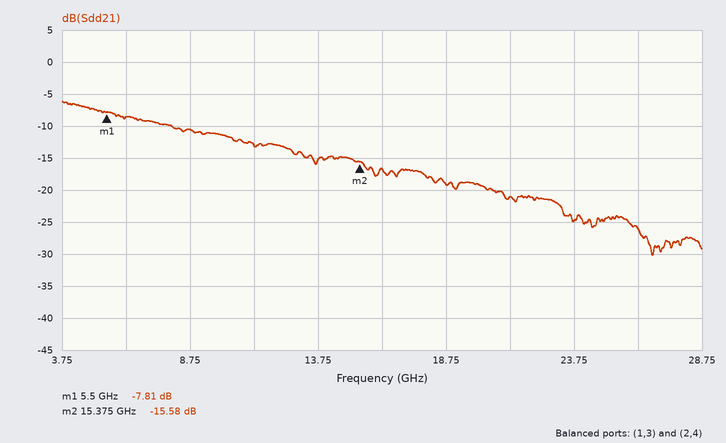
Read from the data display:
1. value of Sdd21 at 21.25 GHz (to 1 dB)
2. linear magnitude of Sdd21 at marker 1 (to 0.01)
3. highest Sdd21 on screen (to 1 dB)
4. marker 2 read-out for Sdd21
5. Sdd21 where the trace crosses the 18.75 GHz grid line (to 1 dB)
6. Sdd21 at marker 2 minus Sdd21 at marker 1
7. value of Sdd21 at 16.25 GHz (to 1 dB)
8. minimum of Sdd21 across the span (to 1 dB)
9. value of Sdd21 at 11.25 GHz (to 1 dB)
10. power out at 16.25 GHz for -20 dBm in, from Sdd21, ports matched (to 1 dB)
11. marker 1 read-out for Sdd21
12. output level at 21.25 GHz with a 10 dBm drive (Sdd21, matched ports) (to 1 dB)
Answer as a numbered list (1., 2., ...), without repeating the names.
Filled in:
1. -21 dB
2. 0.41
3. -6 dB
4. -15.58 dB
5. -19 dB
6. -7.77 dB
7. -17 dB
8. -30 dB
9. -13 dB
10. -37 dBm
11. -7.81 dB
12. -11 dBm
